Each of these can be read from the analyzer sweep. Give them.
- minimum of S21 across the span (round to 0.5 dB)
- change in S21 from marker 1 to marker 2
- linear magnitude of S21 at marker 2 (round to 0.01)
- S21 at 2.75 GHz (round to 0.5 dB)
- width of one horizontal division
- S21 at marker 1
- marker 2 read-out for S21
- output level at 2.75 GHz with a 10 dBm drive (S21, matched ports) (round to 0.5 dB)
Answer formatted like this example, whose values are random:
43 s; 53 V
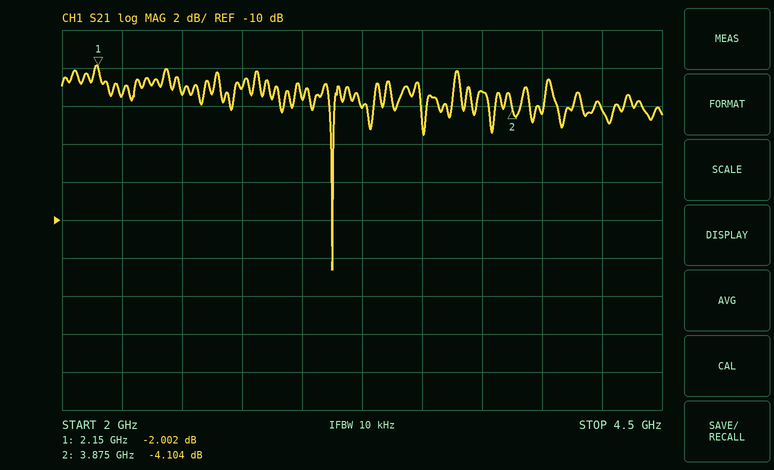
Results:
-12.5 dB; -2.102 dB; 0.62; -3.0 dB; 250 MHz; -2.002 dB; -4.104 dB; 7.0 dBm
